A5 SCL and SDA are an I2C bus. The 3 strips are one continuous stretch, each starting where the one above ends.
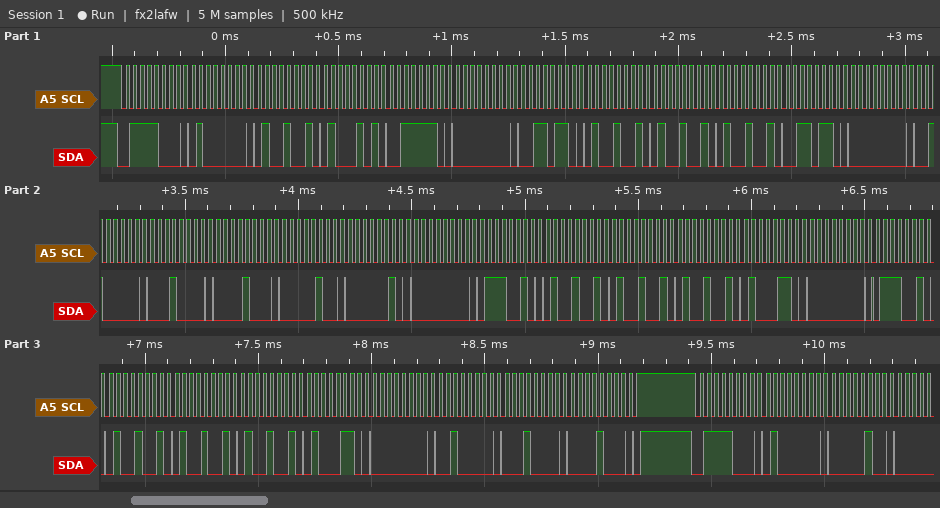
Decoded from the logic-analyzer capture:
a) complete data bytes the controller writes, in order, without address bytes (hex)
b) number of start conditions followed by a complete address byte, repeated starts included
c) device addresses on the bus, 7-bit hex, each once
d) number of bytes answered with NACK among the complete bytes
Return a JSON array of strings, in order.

["40 49 45 3E 00 36 49 49 49 36 00 20 10 08 04 02 00 72 49 49 49 46 00 72 49 49 49 46 00 20 10 08 40 04", "2", "0x3C", "0"]
